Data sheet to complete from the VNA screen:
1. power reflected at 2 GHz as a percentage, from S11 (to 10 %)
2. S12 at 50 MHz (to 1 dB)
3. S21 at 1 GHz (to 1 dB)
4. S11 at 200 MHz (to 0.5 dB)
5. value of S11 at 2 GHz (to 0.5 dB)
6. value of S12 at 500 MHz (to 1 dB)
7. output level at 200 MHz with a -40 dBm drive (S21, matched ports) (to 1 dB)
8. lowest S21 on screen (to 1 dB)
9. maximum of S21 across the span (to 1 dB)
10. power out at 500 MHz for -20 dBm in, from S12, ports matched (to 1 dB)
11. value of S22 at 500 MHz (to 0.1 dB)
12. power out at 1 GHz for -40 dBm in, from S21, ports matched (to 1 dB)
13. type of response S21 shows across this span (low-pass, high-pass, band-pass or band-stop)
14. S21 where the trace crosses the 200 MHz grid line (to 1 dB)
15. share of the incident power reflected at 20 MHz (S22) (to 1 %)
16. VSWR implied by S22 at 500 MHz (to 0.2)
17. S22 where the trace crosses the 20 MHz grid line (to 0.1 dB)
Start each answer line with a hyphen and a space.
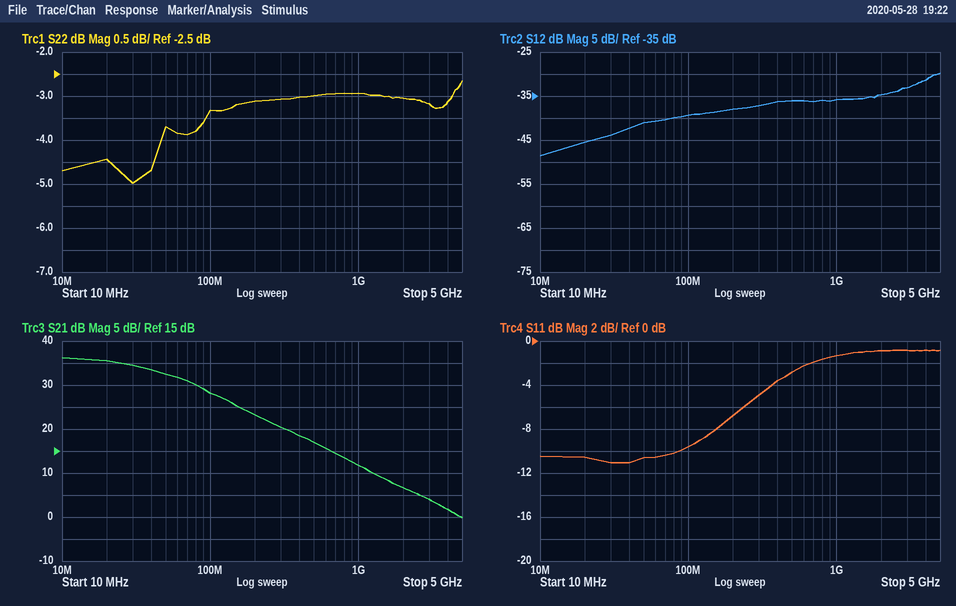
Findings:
- 80 %
- -41 dB
- 12 dB
- -7.0 dB
- -1.0 dB
- -36 dB
- -17 dBm
- 0 dB
- 36 dB
- -56 dBm
- -3.0 dB
- -28 dBm
- low-pass
- 23 dB
- 36 %
- 5.8
- -4.4 dB
